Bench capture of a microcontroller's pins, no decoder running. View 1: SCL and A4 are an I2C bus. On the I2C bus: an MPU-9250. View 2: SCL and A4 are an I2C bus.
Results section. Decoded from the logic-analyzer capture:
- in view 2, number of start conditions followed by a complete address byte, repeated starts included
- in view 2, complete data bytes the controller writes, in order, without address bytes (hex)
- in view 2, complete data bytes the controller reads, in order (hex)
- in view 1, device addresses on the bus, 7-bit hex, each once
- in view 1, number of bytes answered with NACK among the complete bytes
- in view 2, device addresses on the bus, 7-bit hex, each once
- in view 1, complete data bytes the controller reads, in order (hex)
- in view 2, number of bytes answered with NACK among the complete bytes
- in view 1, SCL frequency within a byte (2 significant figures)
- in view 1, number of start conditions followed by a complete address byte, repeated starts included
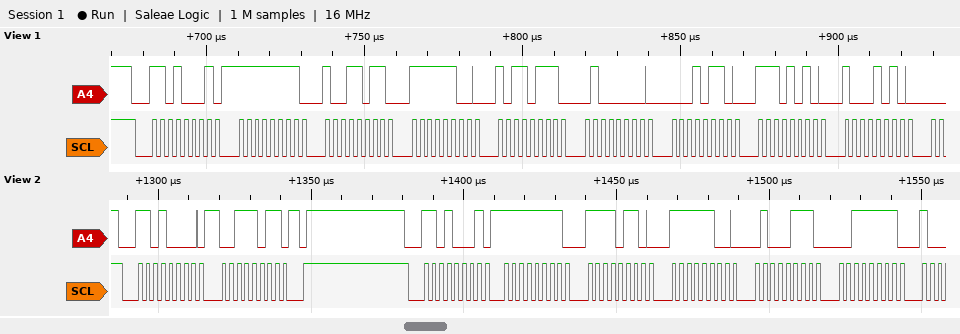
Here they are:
2
3B
FF F6 FC 47 3F
0x68
0
0x68
FF 9B FC B7 40 16 EA 8A
0
400 kHz
1
